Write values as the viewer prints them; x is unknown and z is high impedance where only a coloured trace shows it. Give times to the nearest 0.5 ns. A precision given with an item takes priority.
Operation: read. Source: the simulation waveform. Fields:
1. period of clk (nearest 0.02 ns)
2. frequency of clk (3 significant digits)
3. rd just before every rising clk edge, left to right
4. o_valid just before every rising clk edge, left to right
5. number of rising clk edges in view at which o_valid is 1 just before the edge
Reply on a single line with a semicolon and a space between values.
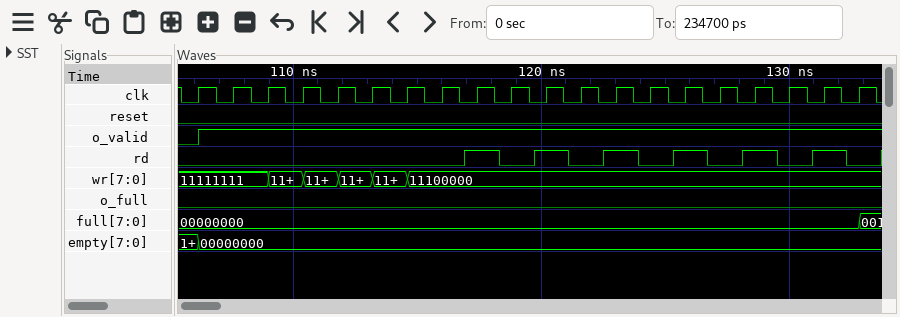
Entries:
1.4 ns; 714 MHz; 0 0 0 0 0 0 0 0 1 0 1 0 1 0 1 0 1 0 1 0; 0 1 1 1 1 1 1 1 1 1 1 1 1 1 1 1 1 1 1 1; 19
